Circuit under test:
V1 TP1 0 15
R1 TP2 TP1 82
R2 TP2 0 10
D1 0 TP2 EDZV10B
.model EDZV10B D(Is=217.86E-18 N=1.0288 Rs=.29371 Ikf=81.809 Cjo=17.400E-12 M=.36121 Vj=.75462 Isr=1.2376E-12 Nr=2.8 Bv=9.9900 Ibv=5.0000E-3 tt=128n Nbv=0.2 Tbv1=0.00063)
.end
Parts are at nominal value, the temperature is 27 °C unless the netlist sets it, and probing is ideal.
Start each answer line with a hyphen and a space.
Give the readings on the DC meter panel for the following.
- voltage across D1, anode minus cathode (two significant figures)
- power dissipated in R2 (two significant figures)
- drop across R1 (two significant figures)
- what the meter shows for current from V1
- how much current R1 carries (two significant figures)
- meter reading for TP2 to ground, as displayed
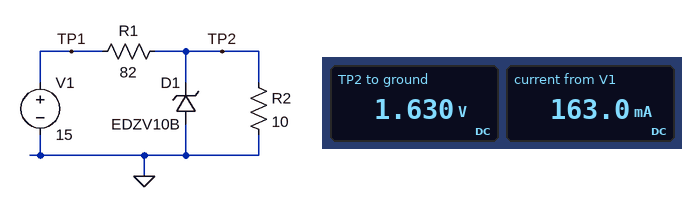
- -1.6 V
- 270 mW
- 13 V
- 163.0 mA
- 160 mA
- 1.630 V
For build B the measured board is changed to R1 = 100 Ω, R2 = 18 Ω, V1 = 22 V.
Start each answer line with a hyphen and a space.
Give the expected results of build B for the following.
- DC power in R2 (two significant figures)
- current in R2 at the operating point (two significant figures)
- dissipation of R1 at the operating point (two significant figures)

- 630 mW
- 190 mA
- 3.5 W
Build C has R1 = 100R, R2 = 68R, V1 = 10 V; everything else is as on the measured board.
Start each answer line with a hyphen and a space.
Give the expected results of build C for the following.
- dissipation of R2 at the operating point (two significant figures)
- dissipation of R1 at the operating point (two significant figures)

- 240 mW
- 350 mW
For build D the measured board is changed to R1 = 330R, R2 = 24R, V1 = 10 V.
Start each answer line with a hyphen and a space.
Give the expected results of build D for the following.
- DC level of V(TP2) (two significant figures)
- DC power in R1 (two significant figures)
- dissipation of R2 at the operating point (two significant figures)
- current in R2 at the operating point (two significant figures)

- 680 mV
- 260 mW
- 19 mW
- 28 mA
